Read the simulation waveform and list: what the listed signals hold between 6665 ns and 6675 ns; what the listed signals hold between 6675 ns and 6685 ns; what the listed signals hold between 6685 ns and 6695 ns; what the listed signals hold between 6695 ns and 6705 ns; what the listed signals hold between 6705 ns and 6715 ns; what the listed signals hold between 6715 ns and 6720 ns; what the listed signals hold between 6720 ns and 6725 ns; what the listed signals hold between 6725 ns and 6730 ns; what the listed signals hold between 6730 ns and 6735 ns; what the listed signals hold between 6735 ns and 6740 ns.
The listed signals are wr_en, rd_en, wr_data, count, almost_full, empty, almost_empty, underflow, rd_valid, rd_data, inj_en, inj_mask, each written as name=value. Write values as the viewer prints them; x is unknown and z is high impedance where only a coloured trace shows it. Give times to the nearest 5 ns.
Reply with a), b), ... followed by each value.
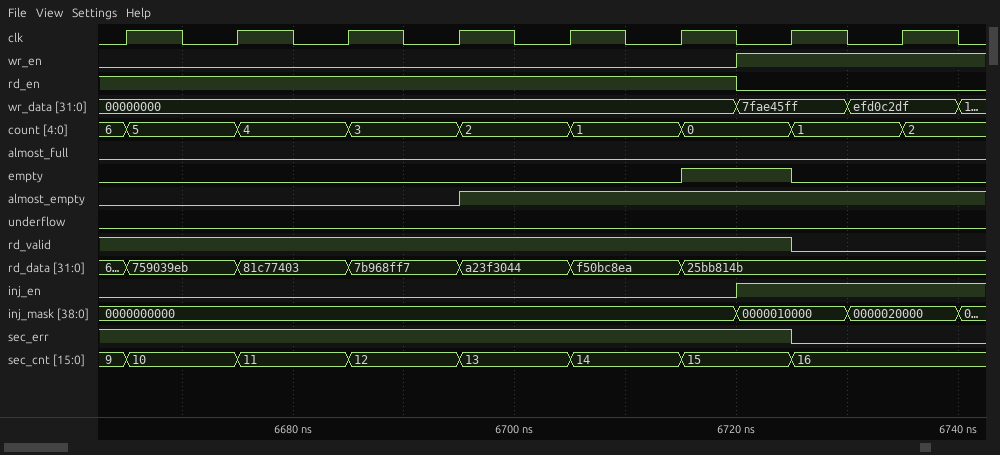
a) wr_en=0, rd_en=1, wr_data=00000000, count=5, almost_full=0, empty=0, almost_empty=0, underflow=0, rd_valid=1, rd_data=759039eb, inj_en=0, inj_mask=0000000000
b) wr_en=0, rd_en=1, wr_data=00000000, count=4, almost_full=0, empty=0, almost_empty=0, underflow=0, rd_valid=1, rd_data=81c77403, inj_en=0, inj_mask=0000000000
c) wr_en=0, rd_en=1, wr_data=00000000, count=3, almost_full=0, empty=0, almost_empty=0, underflow=0, rd_valid=1, rd_data=7b968ff7, inj_en=0, inj_mask=0000000000
d) wr_en=0, rd_en=1, wr_data=00000000, count=2, almost_full=0, empty=0, almost_empty=1, underflow=0, rd_valid=1, rd_data=a23f3044, inj_en=0, inj_mask=0000000000
e) wr_en=0, rd_en=1, wr_data=00000000, count=1, almost_full=0, empty=0, almost_empty=1, underflow=0, rd_valid=1, rd_data=f50bc8ea, inj_en=0, inj_mask=0000000000
f) wr_en=0, rd_en=1, wr_data=00000000, count=0, almost_full=0, empty=1, almost_empty=1, underflow=0, rd_valid=1, rd_data=25bb814b, inj_en=0, inj_mask=0000000000
g) wr_en=1, rd_en=0, wr_data=7fae45ff, count=0, almost_full=0, empty=1, almost_empty=1, underflow=0, rd_valid=1, rd_data=25bb814b, inj_en=1, inj_mask=0000010000
h) wr_en=1, rd_en=0, wr_data=7fae45ff, count=1, almost_full=0, empty=0, almost_empty=1, underflow=0, rd_valid=0, rd_data=25bb814b, inj_en=1, inj_mask=0000010000
i) wr_en=1, rd_en=0, wr_data=efd0c2df, count=1, almost_full=0, empty=0, almost_empty=1, underflow=0, rd_valid=0, rd_data=25bb814b, inj_en=1, inj_mask=0000020000
j) wr_en=1, rd_en=0, wr_data=efd0c2df, count=2, almost_full=0, empty=0, almost_empty=1, underflow=0, rd_valid=0, rd_data=25bb814b, inj_en=1, inj_mask=0000020000
